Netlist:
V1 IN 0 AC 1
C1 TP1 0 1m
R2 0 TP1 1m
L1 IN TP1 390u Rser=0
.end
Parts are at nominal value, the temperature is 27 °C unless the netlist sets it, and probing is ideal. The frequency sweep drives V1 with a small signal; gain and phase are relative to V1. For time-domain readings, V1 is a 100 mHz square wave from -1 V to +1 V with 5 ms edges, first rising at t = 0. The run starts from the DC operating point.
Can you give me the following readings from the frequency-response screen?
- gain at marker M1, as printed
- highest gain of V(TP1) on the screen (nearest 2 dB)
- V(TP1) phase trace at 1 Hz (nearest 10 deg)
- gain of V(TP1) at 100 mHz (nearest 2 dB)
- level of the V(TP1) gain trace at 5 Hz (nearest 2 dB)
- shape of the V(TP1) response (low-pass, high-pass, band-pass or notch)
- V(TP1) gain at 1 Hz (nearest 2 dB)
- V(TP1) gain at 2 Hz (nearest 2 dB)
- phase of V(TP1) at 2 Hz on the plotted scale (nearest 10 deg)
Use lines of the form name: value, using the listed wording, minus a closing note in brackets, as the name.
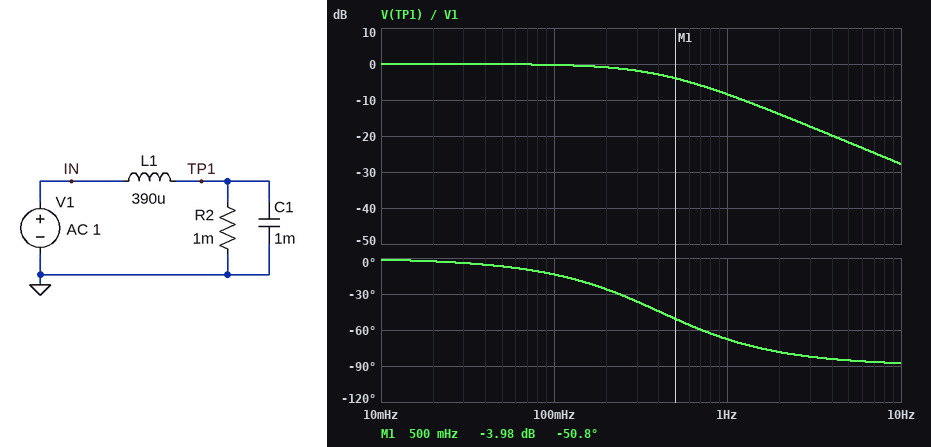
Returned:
gain at marker M1, as printed: -3.98 dB
highest gain of V(TP1) on the screen: 0 dB
V(TP1) phase trace at 1 Hz: -70 deg
gain of V(TP1) at 100 mHz: 0 dB
level of the V(TP1) gain trace at 5 Hz: -22 dB
shape of the V(TP1) response: low-pass
V(TP1) gain at 1 Hz: -8 dB
V(TP1) gain at 2 Hz: -14 dB
phase of V(TP1) at 2 Hz on the plotted scale: -80 deg
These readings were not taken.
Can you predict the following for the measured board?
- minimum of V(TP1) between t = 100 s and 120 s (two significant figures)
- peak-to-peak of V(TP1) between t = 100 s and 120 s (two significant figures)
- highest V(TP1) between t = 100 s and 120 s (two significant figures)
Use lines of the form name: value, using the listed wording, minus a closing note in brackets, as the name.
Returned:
minimum of V(TP1) between t = 100 s and 120 s: -1.0 V
peak-to-peak of V(TP1) between t = 100 s and 120 s: 2.0 V
highest V(TP1) between t = 100 s and 120 s: 1.0 V
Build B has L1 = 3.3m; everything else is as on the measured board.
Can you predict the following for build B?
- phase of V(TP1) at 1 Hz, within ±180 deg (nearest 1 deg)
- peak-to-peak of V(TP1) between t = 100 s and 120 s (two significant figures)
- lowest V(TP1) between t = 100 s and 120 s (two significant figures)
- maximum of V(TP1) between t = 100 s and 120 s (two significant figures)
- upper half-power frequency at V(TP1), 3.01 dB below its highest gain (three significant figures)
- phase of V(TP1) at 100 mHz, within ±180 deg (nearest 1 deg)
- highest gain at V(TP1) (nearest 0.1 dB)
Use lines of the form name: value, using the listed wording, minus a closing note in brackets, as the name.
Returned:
phase of V(TP1) at 1 Hz, within ±180 deg: -87 deg
peak-to-peak of V(TP1) between t = 100 s and 120 s: 1.3 V
lowest V(TP1) between t = 100 s and 120 s: -640 mV
maximum of V(TP1) between t = 100 s and 120 s: 640 mV
upper half-power frequency at V(TP1), 3.01 dB below its highest gain: 48.2 mHz
phase of V(TP1) at 100 mHz, within ±180 deg: -64 deg
highest gain at V(TP1): 0 dB
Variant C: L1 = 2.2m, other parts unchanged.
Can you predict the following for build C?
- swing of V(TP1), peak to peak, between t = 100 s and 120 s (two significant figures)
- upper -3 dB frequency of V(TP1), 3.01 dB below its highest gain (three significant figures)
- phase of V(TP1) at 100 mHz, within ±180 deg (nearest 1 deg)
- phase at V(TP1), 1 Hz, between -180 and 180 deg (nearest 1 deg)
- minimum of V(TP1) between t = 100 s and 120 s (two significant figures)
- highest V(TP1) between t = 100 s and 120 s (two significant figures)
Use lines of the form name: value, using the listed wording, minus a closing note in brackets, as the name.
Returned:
swing of V(TP1), peak to peak, between t = 100 s and 120 s: 1.6 V
upper -3 dB frequency of V(TP1), 3.01 dB below its highest gain: 72.3 mHz
phase of V(TP1) at 100 mHz, within ±180 deg: -54 deg
phase at V(TP1), 1 Hz, between -180 and 180 deg: -86 deg
minimum of V(TP1) between t = 100 s and 120 s: -810 mV
highest V(TP1) between t = 100 s and 120 s: 810 mV
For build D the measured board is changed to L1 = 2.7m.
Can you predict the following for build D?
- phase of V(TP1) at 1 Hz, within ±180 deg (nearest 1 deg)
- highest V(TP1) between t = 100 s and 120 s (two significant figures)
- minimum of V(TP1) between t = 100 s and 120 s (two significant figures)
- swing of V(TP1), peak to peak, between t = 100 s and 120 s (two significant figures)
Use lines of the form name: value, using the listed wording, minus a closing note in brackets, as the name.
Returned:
phase of V(TP1) at 1 Hz, within ±180 deg: -87 deg
highest V(TP1) between t = 100 s and 120 s: 730 mV
minimum of V(TP1) between t = 100 s and 120 s: -730 mV
swing of V(TP1), peak to peak, between t = 100 s and 120 s: 1.5 V
